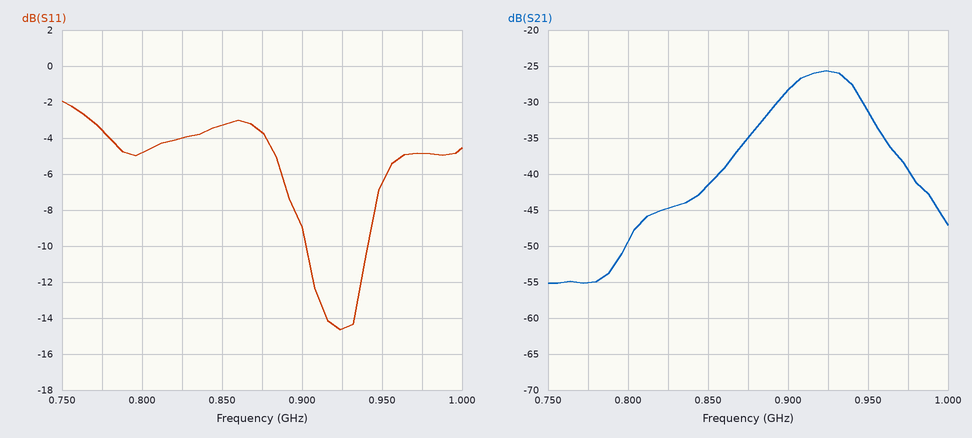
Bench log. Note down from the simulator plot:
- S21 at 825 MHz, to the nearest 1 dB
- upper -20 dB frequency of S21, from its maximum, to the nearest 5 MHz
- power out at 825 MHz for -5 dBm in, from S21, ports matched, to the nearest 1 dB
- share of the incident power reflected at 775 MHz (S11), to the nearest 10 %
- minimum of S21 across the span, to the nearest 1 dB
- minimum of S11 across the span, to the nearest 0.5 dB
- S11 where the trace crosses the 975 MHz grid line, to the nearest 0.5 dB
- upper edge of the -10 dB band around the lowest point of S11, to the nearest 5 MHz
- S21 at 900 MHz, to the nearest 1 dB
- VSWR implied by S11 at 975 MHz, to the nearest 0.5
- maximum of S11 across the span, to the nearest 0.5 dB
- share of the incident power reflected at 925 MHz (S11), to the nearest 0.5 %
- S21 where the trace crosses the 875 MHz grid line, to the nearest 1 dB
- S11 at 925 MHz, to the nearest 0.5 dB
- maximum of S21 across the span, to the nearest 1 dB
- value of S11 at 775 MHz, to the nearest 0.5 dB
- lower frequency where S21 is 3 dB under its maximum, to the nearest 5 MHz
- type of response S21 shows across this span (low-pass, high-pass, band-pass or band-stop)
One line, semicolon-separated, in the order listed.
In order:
-45 dB; 995 MHz; -50 dBm; 40 %; -55 dB; -14.5 dB; -5.0 dB; 940 MHz; -28 dB; 3.5; -2.0 dB; 3.5 %; -35 dB; -14.5 dB; -26 dB; -3.5 dB; 900 MHz; band-pass
